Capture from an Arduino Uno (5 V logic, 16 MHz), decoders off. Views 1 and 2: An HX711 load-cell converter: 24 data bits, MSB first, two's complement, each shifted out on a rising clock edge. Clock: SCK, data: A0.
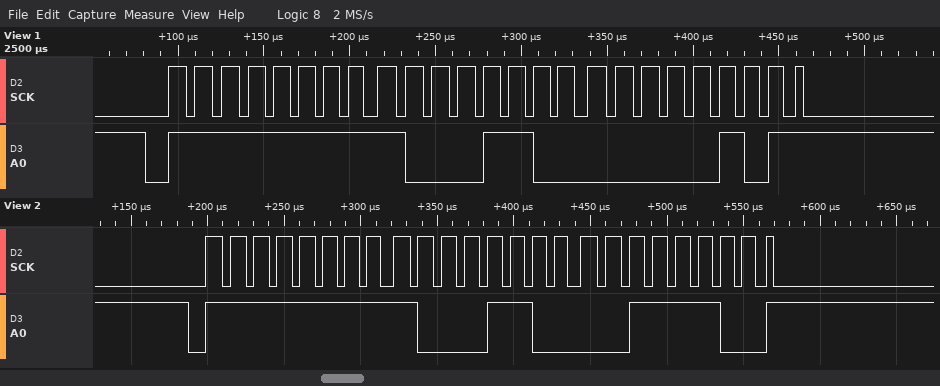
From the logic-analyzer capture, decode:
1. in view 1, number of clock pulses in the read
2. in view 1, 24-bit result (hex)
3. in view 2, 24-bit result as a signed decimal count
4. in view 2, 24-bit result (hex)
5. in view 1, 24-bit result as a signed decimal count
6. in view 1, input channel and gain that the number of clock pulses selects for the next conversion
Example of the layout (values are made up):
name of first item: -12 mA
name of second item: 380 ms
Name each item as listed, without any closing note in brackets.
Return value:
in view 1, number of clock pulses in the read: 25
in view 1, 24-bit result: 0xFF8C05
in view 2, 24-bit result as a signed decimal count: -29636
in view 2, 24-bit result: 0xFF8C3C
in view 1, 24-bit result as a signed decimal count: -29691
in view 1, input channel and gain that the number of clock pulses selects for the next conversion: channel A, gain 128
